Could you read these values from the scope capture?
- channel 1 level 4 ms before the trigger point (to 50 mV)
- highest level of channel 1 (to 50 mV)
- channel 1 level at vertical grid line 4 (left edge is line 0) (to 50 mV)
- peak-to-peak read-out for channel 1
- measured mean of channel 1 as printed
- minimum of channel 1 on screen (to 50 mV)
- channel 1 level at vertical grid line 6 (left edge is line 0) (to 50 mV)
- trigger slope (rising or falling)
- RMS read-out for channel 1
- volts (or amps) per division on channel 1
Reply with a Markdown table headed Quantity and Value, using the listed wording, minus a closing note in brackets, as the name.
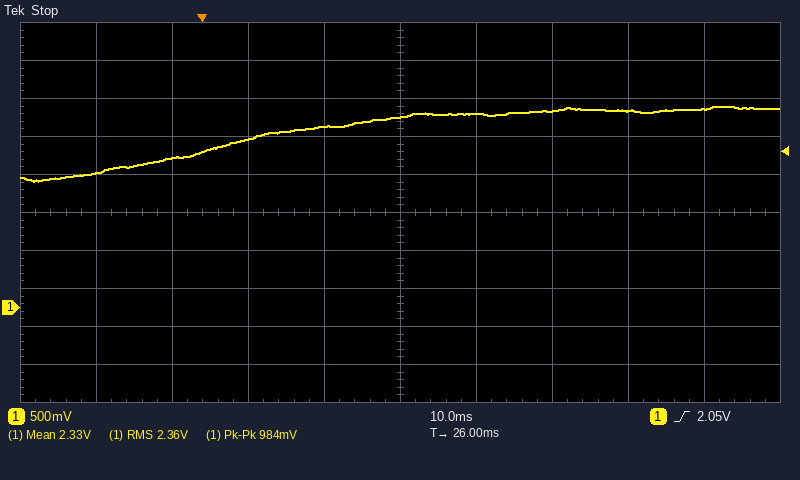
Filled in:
| Quantity | Value |
|---|---|
| channel 1 level 4 ms before the trigger point | 1.95 V |
| highest level of channel 1 | 2.65 V |
| channel 1 level at vertical grid line 4 (left edge is line 0) | 2.40 V |
| peak-to-peak read-out for channel 1 | 984 mV |
| measured mean of channel 1 as printed | 2.33 V |
| minimum of channel 1 on screen | 1.65 V |
| channel 1 level at vertical grid line 6 (left edge is line 0) | 2.55 V |
| trigger slope | rising |
| RMS read-out for channel 1 | 2.36 V |
| volts (or amps) per division on channel 1 | 500 mV |
